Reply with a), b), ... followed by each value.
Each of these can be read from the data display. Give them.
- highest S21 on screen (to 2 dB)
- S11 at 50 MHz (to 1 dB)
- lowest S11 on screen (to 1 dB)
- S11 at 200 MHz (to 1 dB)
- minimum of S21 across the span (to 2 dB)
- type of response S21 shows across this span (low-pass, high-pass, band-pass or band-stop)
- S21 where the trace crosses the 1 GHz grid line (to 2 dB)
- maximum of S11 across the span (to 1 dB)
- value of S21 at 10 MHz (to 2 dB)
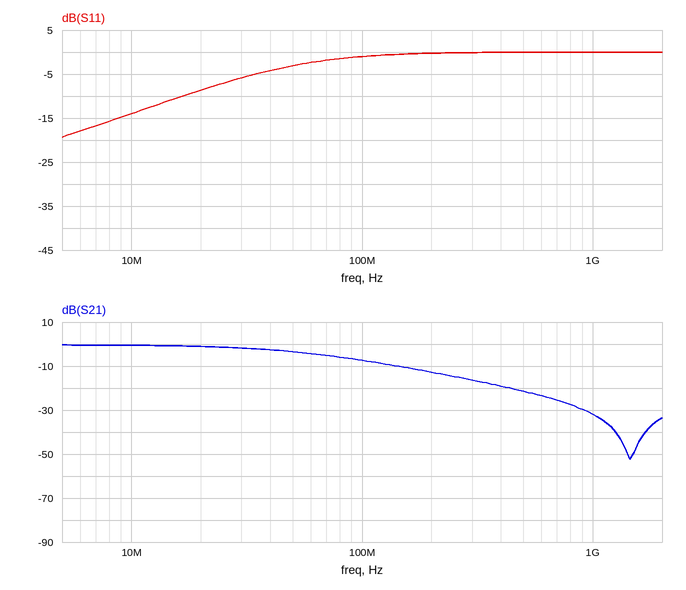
a) 0 dB
b) -3 dB
c) -19 dB
d) 0 dB
e) -52 dB
f) low-pass
g) -32 dB
h) 0 dB
i) 0 dB
